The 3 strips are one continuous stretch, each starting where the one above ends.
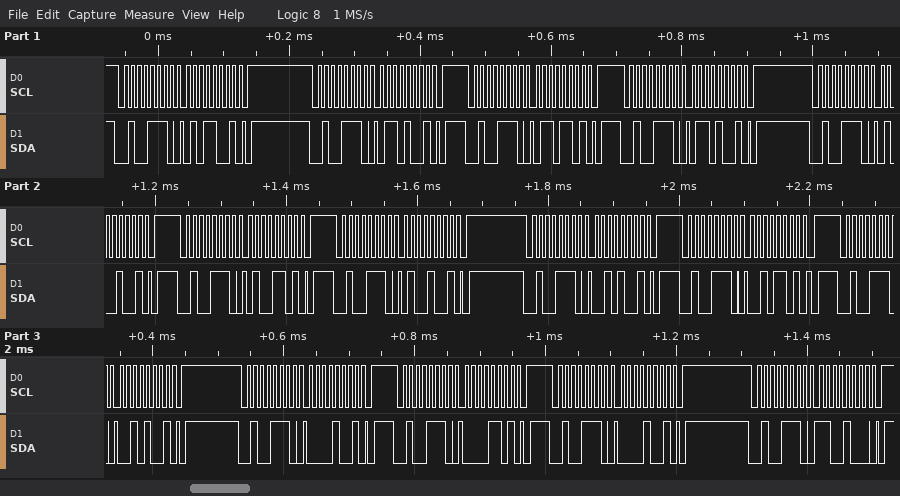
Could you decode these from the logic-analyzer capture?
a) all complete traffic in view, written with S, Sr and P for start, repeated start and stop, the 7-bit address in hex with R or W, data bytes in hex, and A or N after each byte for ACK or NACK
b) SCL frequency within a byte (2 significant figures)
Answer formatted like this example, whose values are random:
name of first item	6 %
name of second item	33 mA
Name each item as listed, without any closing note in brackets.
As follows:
all complete traffic in view, written with S, Sr and P for start, repeated start and stop, the 7-bit address in hex with R or W, data bytes in hex, and A or N after each byte for ACK or NACK	S 27W A 59 A P S 27W A 69 A P S 27W A 6D A P S 27W A 69 A P S 27W A 49 A P S 27W A 4D A P S 27W A 49 A P S 27W A 29 A P S 27W A 2D A P S 27W A 29 A P S 27W A 09 A P S 27W A 0D A P S 27W A 09 A P S 27W A C8 A P
SCL frequency within a byte	100 kHz
